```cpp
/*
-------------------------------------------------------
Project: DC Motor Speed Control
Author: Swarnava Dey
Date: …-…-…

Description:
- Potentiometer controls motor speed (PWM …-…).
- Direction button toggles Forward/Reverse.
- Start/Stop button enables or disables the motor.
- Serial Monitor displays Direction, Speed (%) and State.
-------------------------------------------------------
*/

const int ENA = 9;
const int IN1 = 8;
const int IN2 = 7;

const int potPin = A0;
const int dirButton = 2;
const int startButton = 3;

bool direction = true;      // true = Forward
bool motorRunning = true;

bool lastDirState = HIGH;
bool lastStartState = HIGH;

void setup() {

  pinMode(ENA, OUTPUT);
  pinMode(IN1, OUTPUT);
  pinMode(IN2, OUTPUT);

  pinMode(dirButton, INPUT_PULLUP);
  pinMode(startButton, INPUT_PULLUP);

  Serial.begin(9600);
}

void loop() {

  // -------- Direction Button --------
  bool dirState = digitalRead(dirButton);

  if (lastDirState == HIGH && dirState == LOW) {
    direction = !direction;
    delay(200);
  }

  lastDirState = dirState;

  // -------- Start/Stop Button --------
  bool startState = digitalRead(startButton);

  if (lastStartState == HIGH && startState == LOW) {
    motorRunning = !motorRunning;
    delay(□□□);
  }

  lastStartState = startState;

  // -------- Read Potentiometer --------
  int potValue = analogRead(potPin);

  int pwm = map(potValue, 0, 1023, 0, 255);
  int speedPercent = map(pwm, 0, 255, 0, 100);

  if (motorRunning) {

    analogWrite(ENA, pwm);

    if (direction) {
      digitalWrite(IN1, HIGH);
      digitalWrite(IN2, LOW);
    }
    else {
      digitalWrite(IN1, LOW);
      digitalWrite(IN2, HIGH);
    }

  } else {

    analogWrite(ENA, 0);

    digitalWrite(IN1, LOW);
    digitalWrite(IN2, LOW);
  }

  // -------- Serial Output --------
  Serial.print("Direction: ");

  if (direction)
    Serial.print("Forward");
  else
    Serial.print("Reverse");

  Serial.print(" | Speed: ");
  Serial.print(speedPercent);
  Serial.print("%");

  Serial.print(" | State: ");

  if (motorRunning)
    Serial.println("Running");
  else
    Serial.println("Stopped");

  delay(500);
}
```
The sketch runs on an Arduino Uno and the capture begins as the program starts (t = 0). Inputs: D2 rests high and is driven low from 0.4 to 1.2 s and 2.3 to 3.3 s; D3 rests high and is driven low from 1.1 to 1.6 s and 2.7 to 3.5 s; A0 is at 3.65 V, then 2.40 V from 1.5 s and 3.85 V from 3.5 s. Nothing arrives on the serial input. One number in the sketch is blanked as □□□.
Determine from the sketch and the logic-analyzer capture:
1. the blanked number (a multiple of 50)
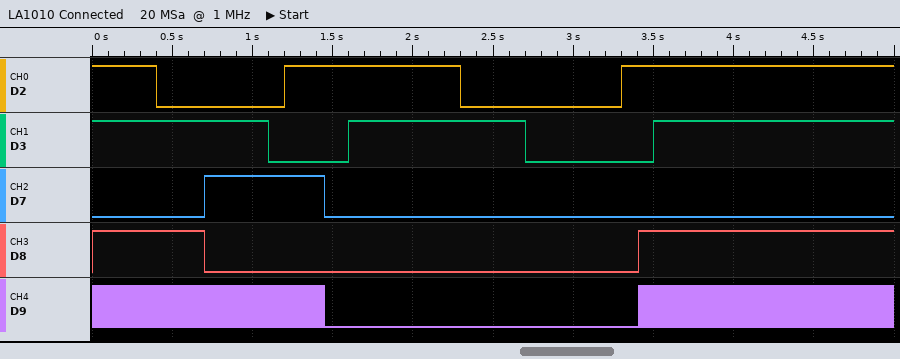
250
